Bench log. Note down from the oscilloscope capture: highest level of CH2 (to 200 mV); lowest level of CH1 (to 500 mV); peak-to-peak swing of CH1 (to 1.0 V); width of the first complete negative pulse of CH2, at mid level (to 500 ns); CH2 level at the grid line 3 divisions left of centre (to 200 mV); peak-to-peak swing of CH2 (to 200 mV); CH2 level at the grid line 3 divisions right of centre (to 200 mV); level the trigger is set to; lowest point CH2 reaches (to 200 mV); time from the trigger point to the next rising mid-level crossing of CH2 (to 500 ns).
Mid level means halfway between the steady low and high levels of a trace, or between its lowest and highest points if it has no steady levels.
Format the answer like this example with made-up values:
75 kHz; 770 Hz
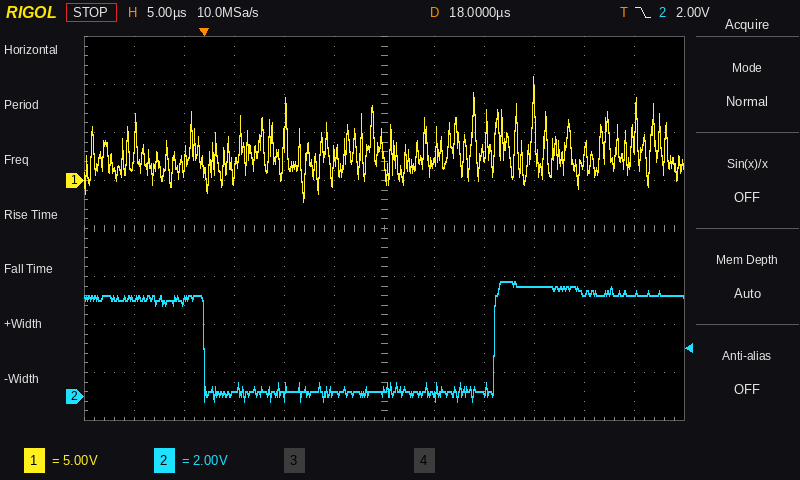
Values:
4.8 V; -2.0 V; 13.0 V; 29.0 µs; 200 mV; 5.0 V; 4.6 V; 2.00 V; -200 mV; 29.0 µs
